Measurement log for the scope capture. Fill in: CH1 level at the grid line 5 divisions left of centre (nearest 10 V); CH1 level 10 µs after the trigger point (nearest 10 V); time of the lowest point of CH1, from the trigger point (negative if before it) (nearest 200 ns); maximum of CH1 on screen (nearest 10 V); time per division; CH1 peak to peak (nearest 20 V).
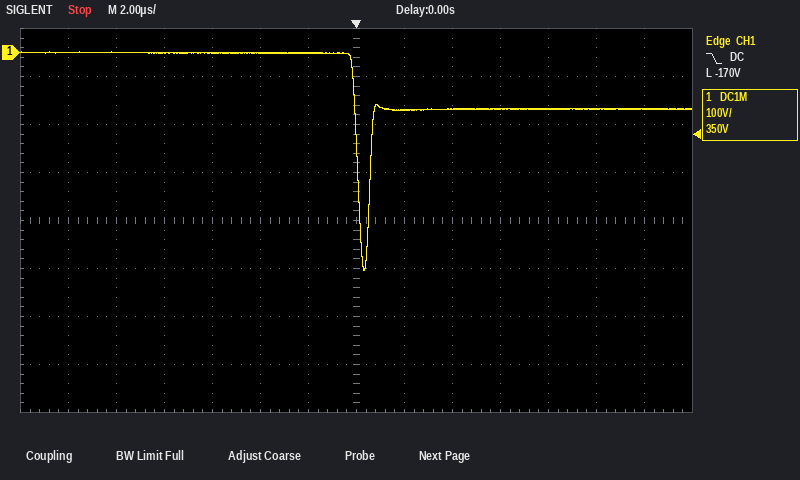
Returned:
0 V
-120 V
+400 ns
0 V
2 µs
460 V
